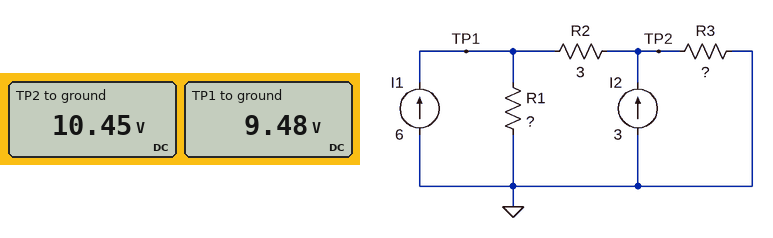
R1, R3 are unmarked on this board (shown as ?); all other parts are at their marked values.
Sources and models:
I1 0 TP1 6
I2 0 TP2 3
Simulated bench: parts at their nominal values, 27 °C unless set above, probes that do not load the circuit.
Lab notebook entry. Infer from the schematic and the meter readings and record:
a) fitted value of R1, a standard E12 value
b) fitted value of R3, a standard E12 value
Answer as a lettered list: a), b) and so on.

a) 1.5 Ω
b) 3.9 Ω
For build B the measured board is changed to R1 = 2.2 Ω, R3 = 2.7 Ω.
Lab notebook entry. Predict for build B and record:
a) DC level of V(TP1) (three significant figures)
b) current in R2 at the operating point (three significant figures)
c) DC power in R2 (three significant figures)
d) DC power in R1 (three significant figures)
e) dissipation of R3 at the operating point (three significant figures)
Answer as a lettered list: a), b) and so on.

a) 11.8 V
b) 646 mA
c) 1.25 W
d) 63.1 W
e) 35.9 W
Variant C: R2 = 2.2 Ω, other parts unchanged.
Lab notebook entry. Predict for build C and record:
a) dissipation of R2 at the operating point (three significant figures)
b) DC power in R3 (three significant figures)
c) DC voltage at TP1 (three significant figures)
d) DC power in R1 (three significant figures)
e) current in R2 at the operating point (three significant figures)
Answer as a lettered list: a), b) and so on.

a) 278 mW
b) 27.3 W
c) 9.53 V
d) 60.6 W
e) 355 mA
